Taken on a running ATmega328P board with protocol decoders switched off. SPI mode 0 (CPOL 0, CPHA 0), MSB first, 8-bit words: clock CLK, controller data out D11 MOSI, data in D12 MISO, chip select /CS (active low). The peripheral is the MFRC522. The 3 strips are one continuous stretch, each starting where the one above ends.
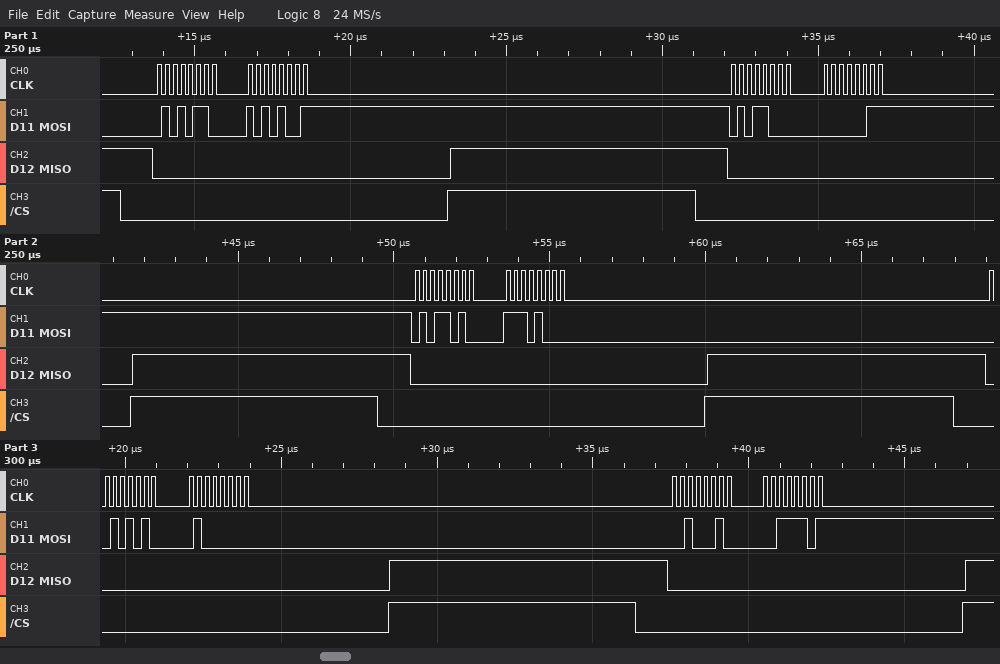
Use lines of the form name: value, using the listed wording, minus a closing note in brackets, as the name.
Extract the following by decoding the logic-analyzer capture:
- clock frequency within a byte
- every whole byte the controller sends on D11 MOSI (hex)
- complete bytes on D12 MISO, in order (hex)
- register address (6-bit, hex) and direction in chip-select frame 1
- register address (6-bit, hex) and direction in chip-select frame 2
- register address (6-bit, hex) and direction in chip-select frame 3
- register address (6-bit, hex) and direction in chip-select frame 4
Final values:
clock frequency within a byte: 4 MHz
every whole byte the controller sends on D11 MOSI: 56 A9 58 03 5A E8 2A 40 22 3D
complete bytes on D12 MISO, in order: 00 00 00 00 00 00 00 00 00 00
register address (6-bit, hex) and direction in chip-select frame 1: 0x2B write
register address (6-bit, hex) and direction in chip-select frame 2: 0x2C write
register address (6-bit, hex) and direction in chip-select frame 3: 0x2D write
register address (6-bit, hex) and direction in chip-select frame 4: 0x15 write
